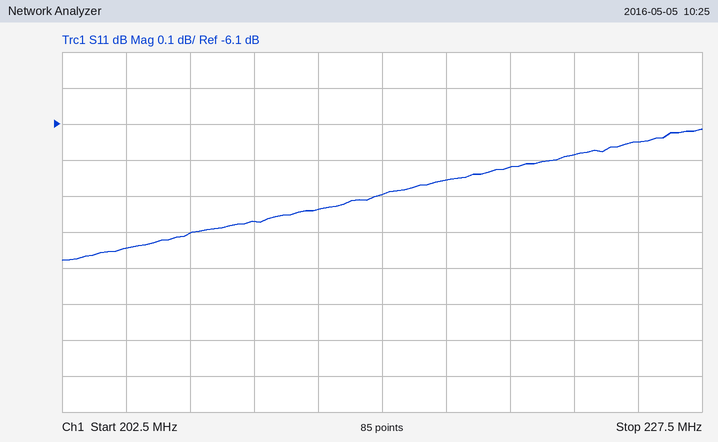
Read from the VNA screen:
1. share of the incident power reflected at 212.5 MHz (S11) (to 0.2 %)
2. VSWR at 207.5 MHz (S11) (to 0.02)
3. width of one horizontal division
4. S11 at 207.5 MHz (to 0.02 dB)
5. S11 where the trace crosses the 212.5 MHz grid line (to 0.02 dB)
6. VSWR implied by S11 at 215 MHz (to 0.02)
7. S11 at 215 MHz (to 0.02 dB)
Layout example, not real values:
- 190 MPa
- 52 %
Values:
- 23.2 %
- 2.84
- 2.5 MHz
- -6.40 dB
- -6.34 dB
- 2.88
- -6.30 dB
